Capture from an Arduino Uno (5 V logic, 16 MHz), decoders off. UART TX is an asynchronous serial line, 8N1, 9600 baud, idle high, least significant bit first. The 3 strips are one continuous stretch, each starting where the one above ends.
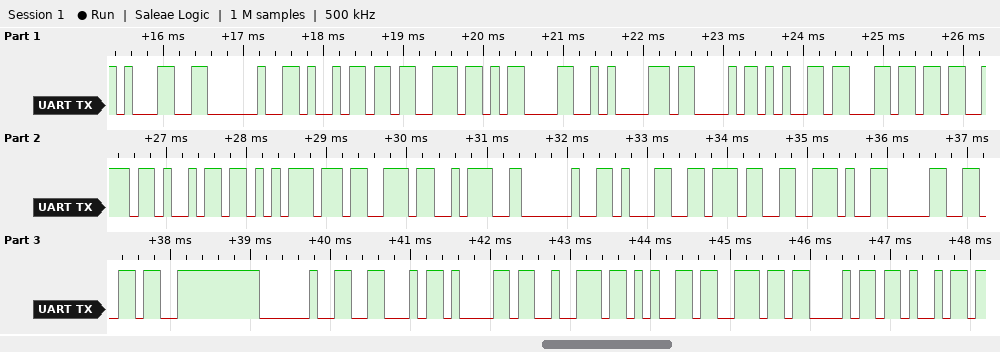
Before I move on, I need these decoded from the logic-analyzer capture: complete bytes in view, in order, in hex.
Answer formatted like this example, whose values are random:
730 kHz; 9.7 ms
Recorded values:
31 20 69 73 0D 0A 43 65 6C 73 69 75 73 3A 20 31 37 2E 30 36 20 46 61 72 65 6E 68 69
